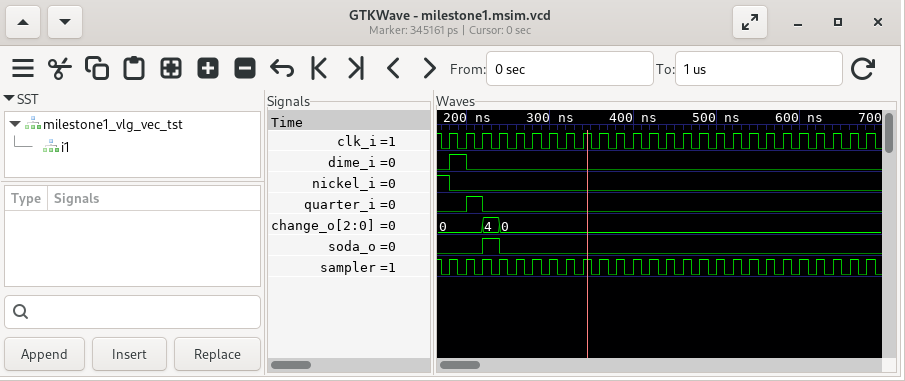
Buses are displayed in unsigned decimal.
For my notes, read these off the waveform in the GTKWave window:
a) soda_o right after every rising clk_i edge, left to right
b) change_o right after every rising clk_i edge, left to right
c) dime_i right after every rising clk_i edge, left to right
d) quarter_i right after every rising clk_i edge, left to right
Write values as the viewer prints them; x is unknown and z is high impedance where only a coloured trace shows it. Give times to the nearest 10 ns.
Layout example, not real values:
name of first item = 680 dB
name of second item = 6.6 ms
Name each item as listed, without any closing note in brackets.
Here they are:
soda_o right after every rising clk_i edge, left to right = 0 0 1 0 0 0 0 0 0 0 0 0 0 0 0 0 0 0 0 0 0 0 0 0 0 0
change_o right after every rising clk_i edge, left to right = 0, 0, 4, 0, 0, 0, 0, 0, 0, 0, 0, 0, 0, 0, 0, 0, 0, 0, 0, 0, 0, 0, 0, 0, 0, 0
dime_i right after every rising clk_i edge, left to right = 1 0 0 0 0 0 0 0 0 0 0 0 0 0 0 0 0 0 0 0 0 0 0 0 0 0
quarter_i right after every rising clk_i edge, left to right = 0 1 0 0 0 0 0 0 0 0 0 0 0 0 0 0 0 0 0 0 0 0 0 0 0 0
